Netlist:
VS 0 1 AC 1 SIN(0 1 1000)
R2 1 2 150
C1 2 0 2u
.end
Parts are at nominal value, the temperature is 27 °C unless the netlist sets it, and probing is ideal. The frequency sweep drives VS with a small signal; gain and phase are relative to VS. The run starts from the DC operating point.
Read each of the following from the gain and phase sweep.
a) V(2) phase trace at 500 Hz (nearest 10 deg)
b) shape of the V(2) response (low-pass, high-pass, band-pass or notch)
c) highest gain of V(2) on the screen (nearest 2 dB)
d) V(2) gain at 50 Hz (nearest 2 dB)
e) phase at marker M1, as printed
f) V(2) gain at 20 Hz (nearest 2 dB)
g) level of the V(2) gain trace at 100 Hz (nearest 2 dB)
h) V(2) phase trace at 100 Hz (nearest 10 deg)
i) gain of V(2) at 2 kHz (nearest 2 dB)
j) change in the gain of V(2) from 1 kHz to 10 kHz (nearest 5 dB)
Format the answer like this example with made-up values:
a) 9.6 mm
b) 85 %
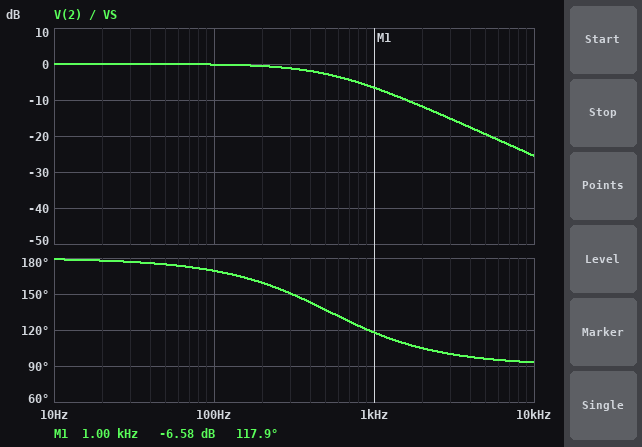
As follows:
a) 140 deg
b) low-pass
c) 0 dB
d) 0 dB
e) 117.9 deg
f) 0 dB
g) 0 dB
h) 170 deg
i) -12 dB
j) -20 dB
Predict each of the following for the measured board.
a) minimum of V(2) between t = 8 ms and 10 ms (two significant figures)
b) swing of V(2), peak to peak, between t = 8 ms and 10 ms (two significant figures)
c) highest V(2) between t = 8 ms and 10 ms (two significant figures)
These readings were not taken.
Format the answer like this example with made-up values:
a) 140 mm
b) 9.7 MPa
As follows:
a) -470 mV
b) 940 mV
c) 470 mV
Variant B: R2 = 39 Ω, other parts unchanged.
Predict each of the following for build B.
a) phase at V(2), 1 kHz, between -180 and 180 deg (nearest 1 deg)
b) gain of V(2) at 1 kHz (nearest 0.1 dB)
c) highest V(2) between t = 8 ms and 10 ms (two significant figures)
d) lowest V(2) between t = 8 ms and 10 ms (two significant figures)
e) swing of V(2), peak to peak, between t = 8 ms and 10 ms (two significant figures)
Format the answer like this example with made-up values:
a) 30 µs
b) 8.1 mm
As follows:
a) 154 deg
b) -0.9 dB
c) 900 mV
d) -900 mV
e) 1.8 V
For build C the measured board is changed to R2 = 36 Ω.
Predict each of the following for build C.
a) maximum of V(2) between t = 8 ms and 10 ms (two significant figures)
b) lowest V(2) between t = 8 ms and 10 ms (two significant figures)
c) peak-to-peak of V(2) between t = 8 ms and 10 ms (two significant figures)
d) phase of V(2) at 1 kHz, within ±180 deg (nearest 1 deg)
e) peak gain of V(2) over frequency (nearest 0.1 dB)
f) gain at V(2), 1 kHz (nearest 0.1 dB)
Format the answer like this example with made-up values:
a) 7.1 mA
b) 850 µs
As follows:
a) 910 mV
b) -910 mV
c) 1.8 V
d) 156 deg
e) 0 dB
f) -0.8 dB
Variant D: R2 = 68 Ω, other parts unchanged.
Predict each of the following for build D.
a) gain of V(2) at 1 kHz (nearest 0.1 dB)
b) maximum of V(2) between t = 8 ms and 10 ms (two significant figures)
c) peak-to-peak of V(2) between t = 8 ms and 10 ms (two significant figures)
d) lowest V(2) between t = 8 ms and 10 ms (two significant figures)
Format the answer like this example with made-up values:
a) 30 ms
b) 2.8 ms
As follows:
a) -2.4 dB
b) 760 mV
c) 1.5 V
d) -760 mV
